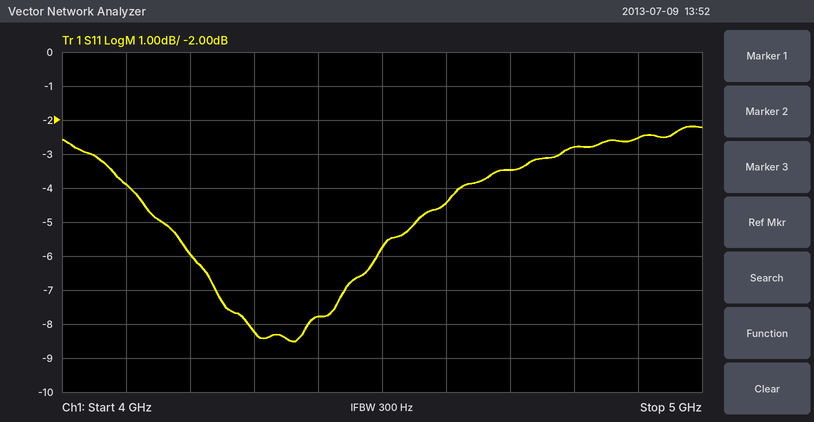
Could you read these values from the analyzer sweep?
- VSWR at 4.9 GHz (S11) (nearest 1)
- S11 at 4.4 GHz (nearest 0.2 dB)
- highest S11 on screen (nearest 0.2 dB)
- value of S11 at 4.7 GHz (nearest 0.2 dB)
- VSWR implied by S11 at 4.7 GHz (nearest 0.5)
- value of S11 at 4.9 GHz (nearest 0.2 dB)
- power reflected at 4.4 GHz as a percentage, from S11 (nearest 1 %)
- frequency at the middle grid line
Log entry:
7
-7.8 dB
-2.2 dB
-3.4 dB
5.0
-2.6 dB
17 %
4.5 GHz
